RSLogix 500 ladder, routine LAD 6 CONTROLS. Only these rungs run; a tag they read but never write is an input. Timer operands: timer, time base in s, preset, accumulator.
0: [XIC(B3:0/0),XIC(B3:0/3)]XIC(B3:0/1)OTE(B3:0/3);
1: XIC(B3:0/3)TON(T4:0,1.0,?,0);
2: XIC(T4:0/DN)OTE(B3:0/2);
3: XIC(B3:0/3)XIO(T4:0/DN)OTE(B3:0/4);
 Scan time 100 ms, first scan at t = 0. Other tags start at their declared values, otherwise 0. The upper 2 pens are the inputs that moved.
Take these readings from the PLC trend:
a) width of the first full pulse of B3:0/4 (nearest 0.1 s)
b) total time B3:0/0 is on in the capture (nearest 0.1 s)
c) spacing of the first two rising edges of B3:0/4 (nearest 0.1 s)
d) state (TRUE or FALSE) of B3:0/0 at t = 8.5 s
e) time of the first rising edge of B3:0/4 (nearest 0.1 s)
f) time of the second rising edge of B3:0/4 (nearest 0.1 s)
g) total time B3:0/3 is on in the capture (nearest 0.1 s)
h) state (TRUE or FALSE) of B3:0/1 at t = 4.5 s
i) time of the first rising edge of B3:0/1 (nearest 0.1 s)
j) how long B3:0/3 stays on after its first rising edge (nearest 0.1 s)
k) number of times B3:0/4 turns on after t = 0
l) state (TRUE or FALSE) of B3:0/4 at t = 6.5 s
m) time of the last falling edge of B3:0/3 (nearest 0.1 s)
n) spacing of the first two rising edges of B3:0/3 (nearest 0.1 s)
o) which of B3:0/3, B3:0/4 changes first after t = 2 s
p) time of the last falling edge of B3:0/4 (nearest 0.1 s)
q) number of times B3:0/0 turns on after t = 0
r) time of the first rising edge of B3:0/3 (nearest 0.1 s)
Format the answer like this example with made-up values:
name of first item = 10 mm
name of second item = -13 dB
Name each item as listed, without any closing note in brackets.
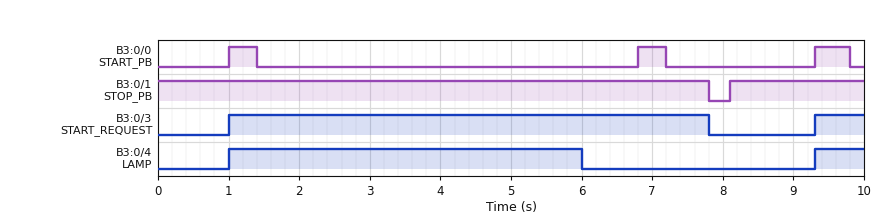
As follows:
width of the first full pulse of B3:0/4 = 5.0 s
total time B3:0/0 is on in the capture = 1.3 s
spacing of the first two rising edges of B3:0/4 = 8.3 s
state (TRUE or FALSE) of B3:0/0 at t = 8.5 s = FALSE
time of the first rising edge of B3:0/4 = 1.0 s
time of the second rising edge of B3:0/4 = 9.3 s
total time B3:0/3 is on in the capture = 7.5 s
state (TRUE or FALSE) of B3:0/1 at t = 4.5 s = TRUE
time of the first rising edge of B3:0/1 = 8.1 s
how long B3:0/3 stays on after its first rising edge = 6.8 s
number of times B3:0/4 turns on after t = 0 = 2
state (TRUE or FALSE) of B3:0/4 at t = 6.5 s = FALSE
time of the last falling edge of B3:0/3 = 7.8 s
spacing of the first two rising edges of B3:0/3 = 8.3 s
which of B3:0/3, B3:0/4 changes first after t = 2 s = B3:0/4
time of the last falling edge of B3:0/4 = 6.0 s
number of times B3:0/0 turns on after t = 0 = 3
time of the first rising edge of B3:0/3 = 1.0 s
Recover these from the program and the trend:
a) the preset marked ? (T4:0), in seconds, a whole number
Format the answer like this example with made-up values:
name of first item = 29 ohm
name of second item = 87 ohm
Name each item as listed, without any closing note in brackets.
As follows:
the preset marked ? (T4:0), in seconds, a whole number = 5 s
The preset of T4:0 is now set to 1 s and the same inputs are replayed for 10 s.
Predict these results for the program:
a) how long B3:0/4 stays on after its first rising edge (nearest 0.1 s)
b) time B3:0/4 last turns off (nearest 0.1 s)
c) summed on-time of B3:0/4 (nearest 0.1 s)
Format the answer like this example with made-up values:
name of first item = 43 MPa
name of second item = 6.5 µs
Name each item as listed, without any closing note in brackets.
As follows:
how long B3:0/4 stays on after its first rising edge = 1.0 s
time B3:0/4 last turns off = 2.0 s
summed on-time of B3:0/4 = 1.7 s
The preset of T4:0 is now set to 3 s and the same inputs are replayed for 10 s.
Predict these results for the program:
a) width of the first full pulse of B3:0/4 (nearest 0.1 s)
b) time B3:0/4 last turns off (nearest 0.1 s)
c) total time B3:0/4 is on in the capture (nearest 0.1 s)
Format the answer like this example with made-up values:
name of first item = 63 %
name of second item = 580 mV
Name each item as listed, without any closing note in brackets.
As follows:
width of the first full pulse of B3:0/4 = 3.0 s
time B3:0/4 last turns off = 4.0 s
total time B3:0/4 is on in the capture = 3.7 s
